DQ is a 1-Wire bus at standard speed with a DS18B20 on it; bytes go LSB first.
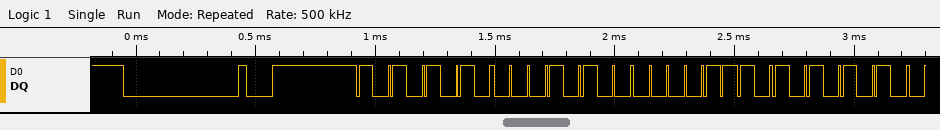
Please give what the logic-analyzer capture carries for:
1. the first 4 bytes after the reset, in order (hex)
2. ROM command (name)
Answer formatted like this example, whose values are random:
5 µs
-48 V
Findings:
55 28 70 55
Match ROM
